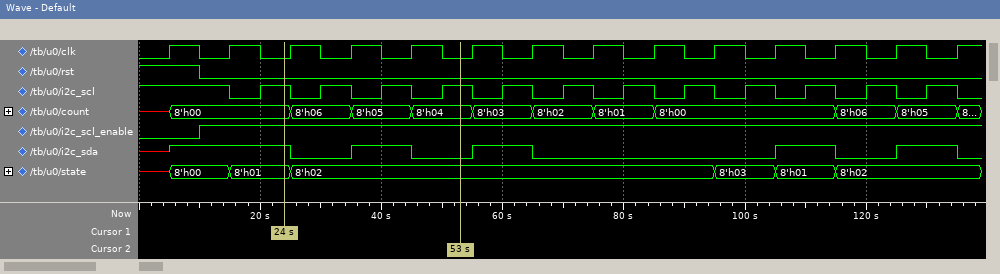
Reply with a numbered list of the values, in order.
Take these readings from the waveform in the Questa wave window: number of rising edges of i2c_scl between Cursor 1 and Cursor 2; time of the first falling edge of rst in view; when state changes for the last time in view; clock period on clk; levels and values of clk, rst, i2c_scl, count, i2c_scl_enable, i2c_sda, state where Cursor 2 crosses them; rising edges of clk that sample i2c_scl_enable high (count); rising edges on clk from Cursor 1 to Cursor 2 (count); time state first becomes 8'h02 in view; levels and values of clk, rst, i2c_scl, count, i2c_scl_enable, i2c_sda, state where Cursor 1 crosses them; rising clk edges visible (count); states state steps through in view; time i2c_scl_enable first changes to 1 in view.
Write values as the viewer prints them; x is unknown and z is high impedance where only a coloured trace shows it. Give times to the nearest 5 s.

1. 3
2. 10 s
3. 115 s
4. 10 s
5. clk=0, rst=0, i2c_scl=1, count=8'h04, i2c_scl_enable=1, i2c_sda=0, state=8'h02
6. 13
7. 3
8. 25 s
9. clk=0, rst=0, i2c_scl=1, count=8'h00, i2c_scl_enable=1, i2c_sda=1, state=8'h01
10. 14
11. x, 8'h00, 8'h01, 8'h02, 8'h03, 8'h01, 8'h02
12. 10 s
